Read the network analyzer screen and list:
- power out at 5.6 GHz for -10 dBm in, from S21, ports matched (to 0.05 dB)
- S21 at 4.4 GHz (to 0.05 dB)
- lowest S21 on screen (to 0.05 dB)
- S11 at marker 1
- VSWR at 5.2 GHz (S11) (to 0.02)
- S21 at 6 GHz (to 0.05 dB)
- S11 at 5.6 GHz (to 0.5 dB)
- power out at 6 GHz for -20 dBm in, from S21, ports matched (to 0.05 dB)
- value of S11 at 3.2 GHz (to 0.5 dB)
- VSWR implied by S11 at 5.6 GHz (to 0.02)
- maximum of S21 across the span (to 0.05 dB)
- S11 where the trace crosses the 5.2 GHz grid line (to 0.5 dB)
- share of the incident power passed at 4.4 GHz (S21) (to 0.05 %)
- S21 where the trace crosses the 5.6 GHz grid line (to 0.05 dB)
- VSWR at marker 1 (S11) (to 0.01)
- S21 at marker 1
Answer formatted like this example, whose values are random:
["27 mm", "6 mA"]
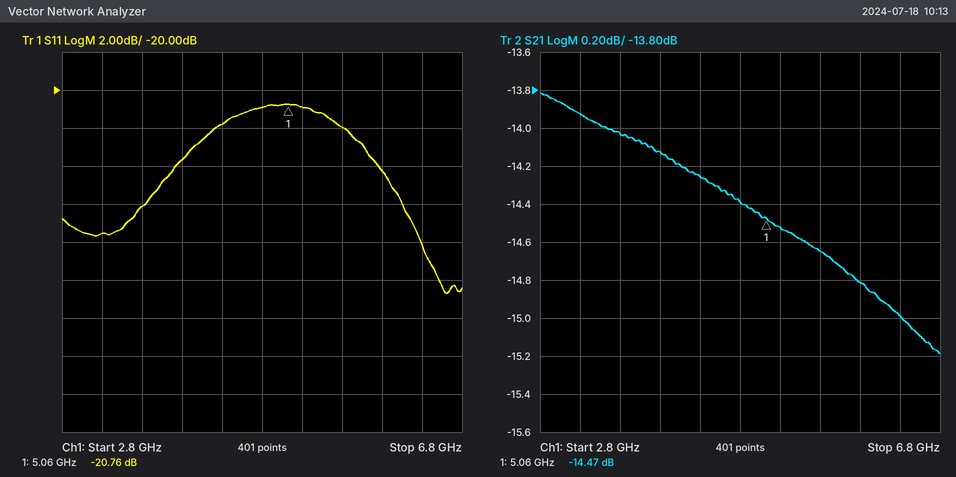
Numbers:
["-24.65 dBm", "-14.25 dB", "-15.20 dB", "-20.76 dB", "1.20", "-14.80 dB", "-22.0 dB", "-34.80 dBm", "-27.5 dB", "1.18", "-13.80 dB", "-21.0 dB", "3.75 %", "-14.65 dB", "1.20", "-14.47 dB"]
